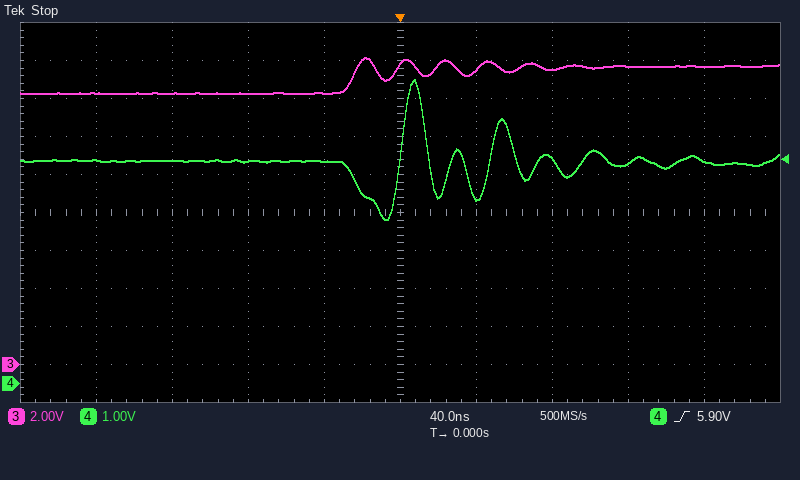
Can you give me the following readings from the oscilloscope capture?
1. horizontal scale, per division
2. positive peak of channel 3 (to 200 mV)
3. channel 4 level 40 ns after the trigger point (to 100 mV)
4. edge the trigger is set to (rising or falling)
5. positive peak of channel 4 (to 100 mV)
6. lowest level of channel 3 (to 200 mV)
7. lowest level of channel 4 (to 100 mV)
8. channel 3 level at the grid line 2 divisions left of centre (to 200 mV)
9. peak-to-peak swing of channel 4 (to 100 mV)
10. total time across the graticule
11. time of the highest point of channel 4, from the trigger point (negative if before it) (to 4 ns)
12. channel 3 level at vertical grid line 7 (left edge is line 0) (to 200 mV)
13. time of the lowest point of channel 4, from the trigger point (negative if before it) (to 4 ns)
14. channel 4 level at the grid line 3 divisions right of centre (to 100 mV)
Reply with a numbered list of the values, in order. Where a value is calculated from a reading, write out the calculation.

1. 40 ns
2. 16.2 V
3. 4.9 V
4. rising
5. 8.0 V
6. 14.2 V
7. 4.3 V
8. 14.2 V
9. 8.0 V − (4.3 V) = 3.7 V
10. 400 ns
11. +8 ns
12. 15.6 V
13. -8 ns
14. 5.8 V
